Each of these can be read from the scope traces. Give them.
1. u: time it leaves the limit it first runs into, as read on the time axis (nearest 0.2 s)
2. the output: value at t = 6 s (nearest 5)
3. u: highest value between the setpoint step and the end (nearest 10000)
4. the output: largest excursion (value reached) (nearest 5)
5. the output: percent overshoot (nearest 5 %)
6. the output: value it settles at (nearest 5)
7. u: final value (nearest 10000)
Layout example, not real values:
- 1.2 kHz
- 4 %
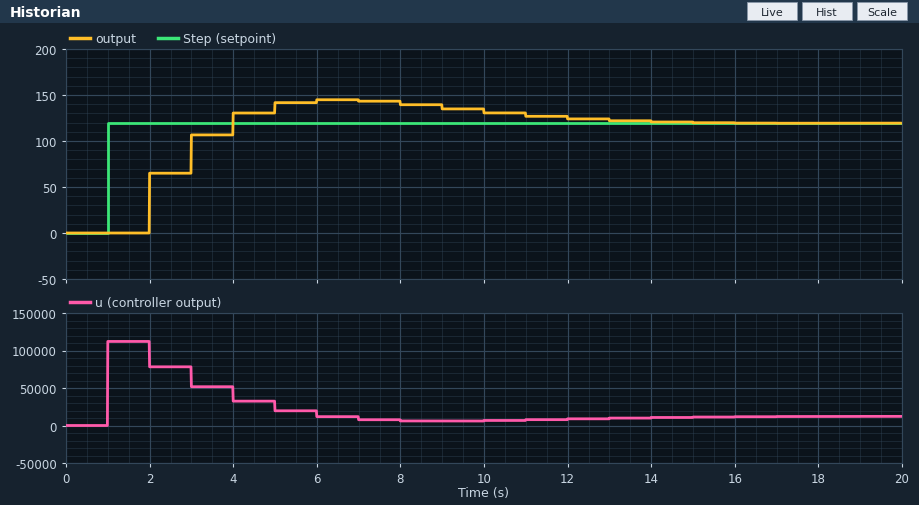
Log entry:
- 2.0 s
- 145
- 110000
- 145
- 20 %
- 120
- 10000
